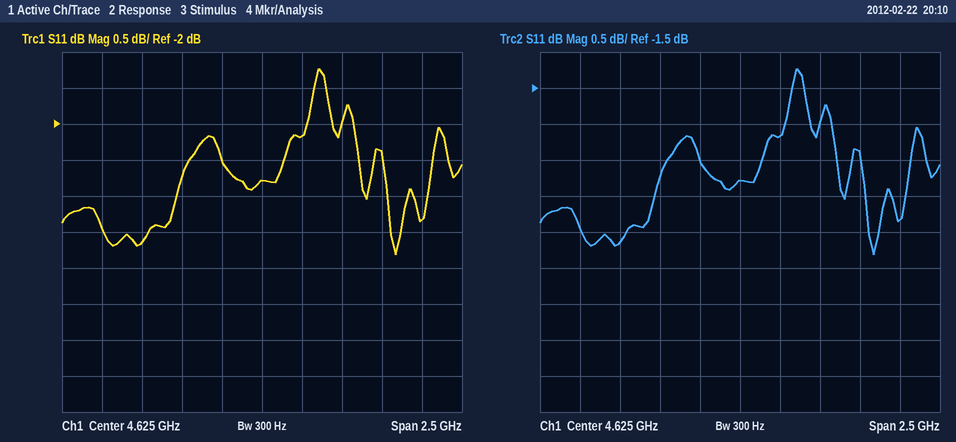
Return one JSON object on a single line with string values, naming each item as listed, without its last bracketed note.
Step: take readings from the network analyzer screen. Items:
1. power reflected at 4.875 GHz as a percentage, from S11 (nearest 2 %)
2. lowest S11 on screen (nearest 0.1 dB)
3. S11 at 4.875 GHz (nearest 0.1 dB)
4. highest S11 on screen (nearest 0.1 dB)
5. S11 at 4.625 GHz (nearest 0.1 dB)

{"power reflected at 4.875 GHz as a percentage, from S11": "60 %", "lowest S11 on screen": "-3.8 dB", "S11 at 4.875 GHz": "-2.2 dB", "highest S11 on screen": "-1.2 dB", "S11 at 4.625 GHz": "-2.8 dB"}
